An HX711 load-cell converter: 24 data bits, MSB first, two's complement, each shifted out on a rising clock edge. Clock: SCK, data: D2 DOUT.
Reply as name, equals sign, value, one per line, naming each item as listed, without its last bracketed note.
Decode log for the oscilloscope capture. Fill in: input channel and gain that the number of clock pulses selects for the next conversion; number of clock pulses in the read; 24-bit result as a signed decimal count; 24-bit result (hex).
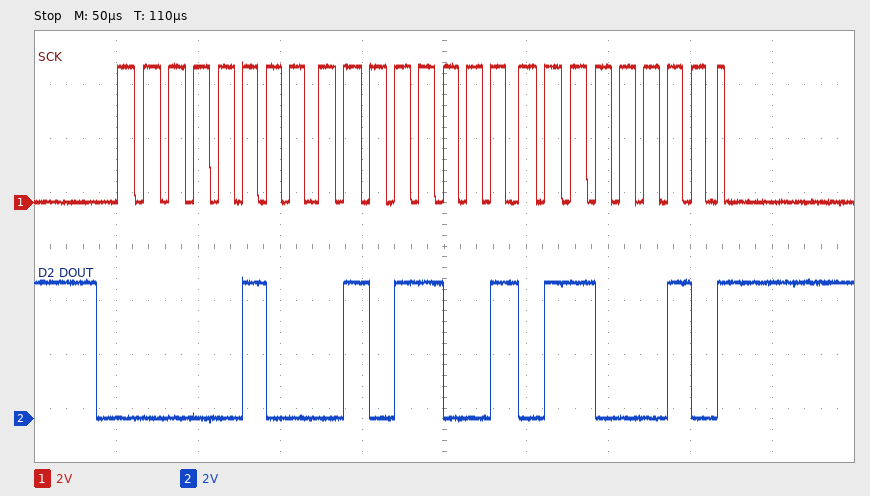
input channel and gain that the number of clock pulses selects for the next conversion = channel A, gain 128
number of clock pulses in the read = 25
24-bit result as a signed decimal count = 285026
24-bit result = 0x045962
